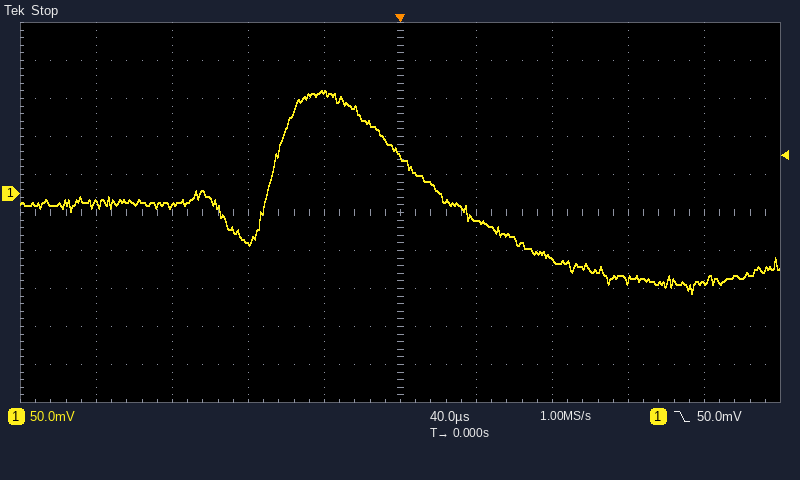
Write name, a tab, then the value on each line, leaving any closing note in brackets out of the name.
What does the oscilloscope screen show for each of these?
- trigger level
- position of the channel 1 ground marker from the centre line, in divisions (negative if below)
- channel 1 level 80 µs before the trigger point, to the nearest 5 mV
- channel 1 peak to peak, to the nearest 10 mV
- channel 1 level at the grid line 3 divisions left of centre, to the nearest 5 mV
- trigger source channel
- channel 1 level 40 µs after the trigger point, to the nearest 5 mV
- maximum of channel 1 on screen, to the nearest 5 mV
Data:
trigger level	50.0 mV
position of the channel 1 ground marker from the centre line, in divisions	+0.5 div
channel 1 level 80 µs before the trigger point, to the nearest 5 mV	-65 mV
channel 1 peak to peak, to the nearest 10 mV	270 mV
channel 1 level at the grid line 3 divisions left of centre, to the nearest 5 mV	-15 mV
trigger source channel	channel 1
channel 1 level 40 µs after the trigger point, to the nearest 5 mV	-35 mV
maximum of channel 1 on screen, to the nearest 5 mV	135 mV
